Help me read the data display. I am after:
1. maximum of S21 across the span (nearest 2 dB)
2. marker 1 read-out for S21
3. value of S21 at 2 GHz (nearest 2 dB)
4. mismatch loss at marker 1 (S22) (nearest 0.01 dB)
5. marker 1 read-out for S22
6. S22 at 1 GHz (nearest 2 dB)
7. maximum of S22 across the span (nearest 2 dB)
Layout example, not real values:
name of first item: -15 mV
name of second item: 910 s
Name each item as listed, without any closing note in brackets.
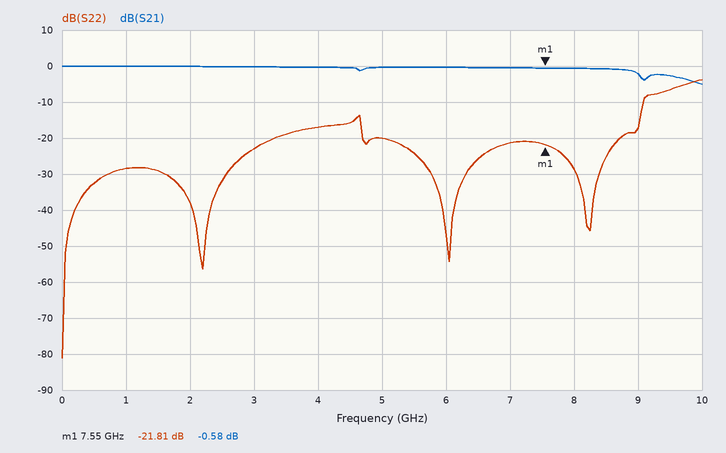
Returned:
maximum of S21 across the span: 0 dB
marker 1 read-out for S21: -0.58 dB
value of S21 at 2 GHz: 0 dB
mismatch loss at marker 1 (S22): 0.03 dB
marker 1 read-out for S22: -21.81 dB
S22 at 1 GHz: -28 dB
maximum of S22 across the span: -4 dB
